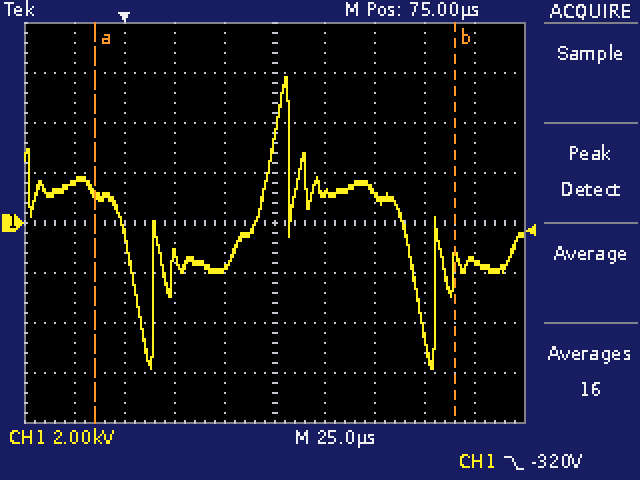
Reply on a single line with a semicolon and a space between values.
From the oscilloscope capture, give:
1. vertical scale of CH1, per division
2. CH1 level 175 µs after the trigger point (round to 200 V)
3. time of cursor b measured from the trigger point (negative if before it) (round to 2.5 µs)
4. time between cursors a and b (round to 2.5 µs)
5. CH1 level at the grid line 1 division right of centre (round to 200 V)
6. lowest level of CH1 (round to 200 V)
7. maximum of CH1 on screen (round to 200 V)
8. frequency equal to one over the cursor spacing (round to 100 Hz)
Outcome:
2 kV; -1.6 kV; +165.0 µs; 180.0 µs; 1.2 kV; -5.8 kV; 5.8 kV; 5.6 kHz
